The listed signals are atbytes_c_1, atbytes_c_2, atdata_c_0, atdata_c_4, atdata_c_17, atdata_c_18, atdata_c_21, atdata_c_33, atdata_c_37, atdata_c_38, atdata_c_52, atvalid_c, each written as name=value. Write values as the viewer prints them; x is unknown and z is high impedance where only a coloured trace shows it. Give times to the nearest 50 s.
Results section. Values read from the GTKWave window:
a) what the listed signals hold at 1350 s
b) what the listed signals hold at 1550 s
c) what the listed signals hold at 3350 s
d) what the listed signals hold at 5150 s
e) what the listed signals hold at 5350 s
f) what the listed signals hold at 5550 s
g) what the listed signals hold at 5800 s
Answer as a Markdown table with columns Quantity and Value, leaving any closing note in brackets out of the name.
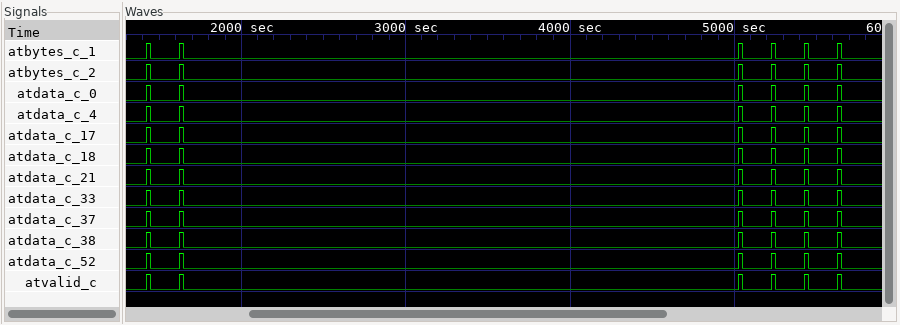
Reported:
| Quantity | Value |
|---|---|
| what the listed signals hold at 1350 s | atbytes_c_1=0, atbytes_c_2=0, atdata_c_0=0, atdata_c_4=0, atdata_c_17=0, atdata_c_18=0, atdata_c_21=0, atdata_c_33=0, atdata_c_37=0, atdata_c_38=0, atdata_c_52=0, atvalid_c=0 |
| what the listed signals hold at 1550 s | atbytes_c_1=0, atbytes_c_2=0, atdata_c_0=0, atdata_c_4=0, atdata_c_17=0, atdata_c_18=0, atdata_c_21=0, atdata_c_33=0, atdata_c_37=0, atdata_c_38=0, atdata_c_52=0, atvalid_c=0 |
| what the listed signals hold at 3350 s | atbytes_c_1=0, atbytes_c_2=0, atdata_c_0=0, atdata_c_4=0, atdata_c_17=0, atdata_c_18=0, atdata_c_21=0, atdata_c_33=0, atdata_c_37=0, atdata_c_38=0, atdata_c_52=0, atvalid_c=0 |
| what the listed signals hold at 5150 s | atbytes_c_1=0, atbytes_c_2=0, atdata_c_0=0, atdata_c_4=0, atdata_c_17=0, atdata_c_18=0, atdata_c_21=0, atdata_c_33=0, atdata_c_37=0, atdata_c_38=0, atdata_c_52=0, atvalid_c=0 |
| what the listed signals hold at 5350 s | atbytes_c_1=0, atbytes_c_2=0, atdata_c_0=0, atdata_c_4=0, atdata_c_17=0, atdata_c_18=0, atdata_c_21=0, atdata_c_33=0, atdata_c_37=0, atdata_c_38=0, atdata_c_52=0, atvalid_c=0 |
| what the listed signals hold at 5550 s | atbytes_c_1=0, atbytes_c_2=0, atdata_c_0=0, atdata_c_4=0, atdata_c_17=0, atdata_c_18=0, atdata_c_21=0, atdata_c_33=0, atdata_c_37=0, atdata_c_38=0, atdata_c_52=0, atvalid_c=0 |
| what the listed signals hold at 5800 s | atbytes_c_1=0, atbytes_c_2=0, atdata_c_0=0, atdata_c_4=0, atdata_c_17=0, atdata_c_18=0, atdata_c_21=0, atdata_c_33=0, atdata_c_37=0, atdata_c_38=0, atdata_c_52=0, atvalid_c=0 |
